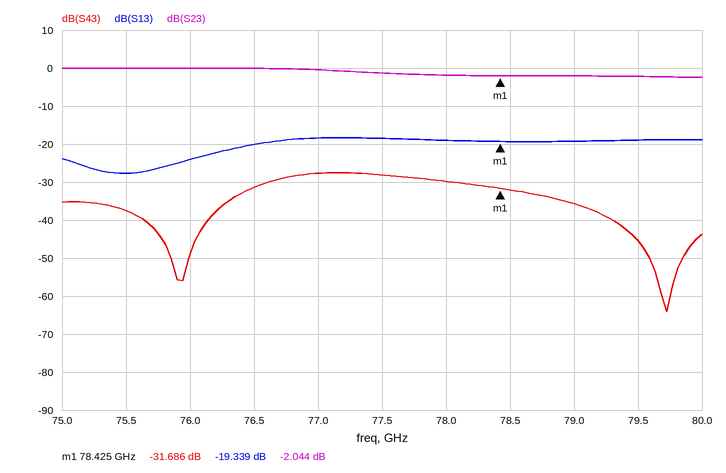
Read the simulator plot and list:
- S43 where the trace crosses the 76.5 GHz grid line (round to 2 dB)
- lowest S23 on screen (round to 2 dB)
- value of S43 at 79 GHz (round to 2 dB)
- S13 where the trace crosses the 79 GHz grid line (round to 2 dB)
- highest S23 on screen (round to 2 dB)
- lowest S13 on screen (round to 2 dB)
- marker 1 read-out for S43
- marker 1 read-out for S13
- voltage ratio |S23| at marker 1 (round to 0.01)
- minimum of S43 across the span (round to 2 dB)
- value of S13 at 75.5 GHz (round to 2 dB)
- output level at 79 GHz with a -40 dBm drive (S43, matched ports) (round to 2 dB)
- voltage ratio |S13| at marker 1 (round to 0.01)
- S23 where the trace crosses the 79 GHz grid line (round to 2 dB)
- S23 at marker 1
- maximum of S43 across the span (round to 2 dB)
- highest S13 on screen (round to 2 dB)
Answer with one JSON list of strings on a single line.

["-32 dB", "-2 dB", "-36 dB", "-20 dB", "0 dB", "-28 dB", "-31.686 dB", "-19.339 dB", "0.79", "-64 dB", "-28 dB", "-76 dBm", "0.11", "-2 dB", "-2.044 dB", "-28 dB", "-18 dB"]
